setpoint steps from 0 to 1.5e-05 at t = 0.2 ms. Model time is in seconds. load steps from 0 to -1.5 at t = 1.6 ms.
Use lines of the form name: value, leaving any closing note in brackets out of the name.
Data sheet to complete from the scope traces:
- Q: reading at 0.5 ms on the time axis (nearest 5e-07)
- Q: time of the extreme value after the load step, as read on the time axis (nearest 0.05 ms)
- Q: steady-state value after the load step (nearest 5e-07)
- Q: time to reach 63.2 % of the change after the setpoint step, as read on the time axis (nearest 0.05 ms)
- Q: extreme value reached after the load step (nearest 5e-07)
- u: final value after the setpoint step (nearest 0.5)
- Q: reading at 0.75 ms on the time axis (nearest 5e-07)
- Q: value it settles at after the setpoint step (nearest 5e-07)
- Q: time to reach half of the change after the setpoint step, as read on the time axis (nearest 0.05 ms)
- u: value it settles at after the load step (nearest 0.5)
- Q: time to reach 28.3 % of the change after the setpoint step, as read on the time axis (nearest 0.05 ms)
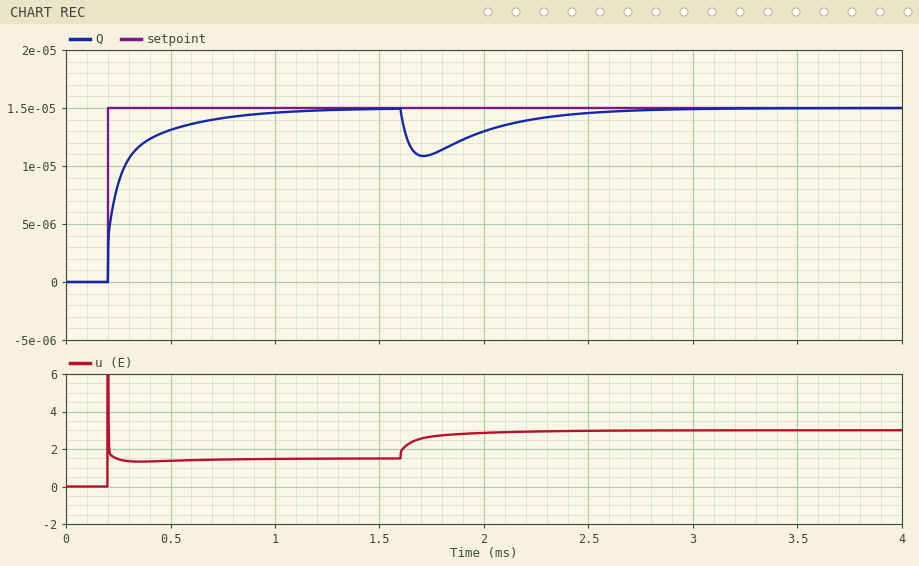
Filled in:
Q: reading at 0.5 ms on the time axis: 0.0000130
Q: time of the extreme value after the load step, as read on the time axis: 1.70 ms
Q: steady-state value after the load step: 0.0000150
Q: time to reach 63.2 % of the change after the setpoint step, as read on the time axis: 0.25 ms
Q: extreme value reached after the load step: 0.0000110
u: final value after the setpoint step: 1.5
Q: reading at 0.75 ms on the time axis: 0.0000140
Q: value it settles at after the setpoint step: 0.0000150
Q: time to reach half of the change after the setpoint step, as read on the time axis: 0.25 ms
u: value it settles at after the load step: 3.0
Q: time to reach 28.3 % of the change after the setpoint step, as read on the time axis: 0.20 ms
